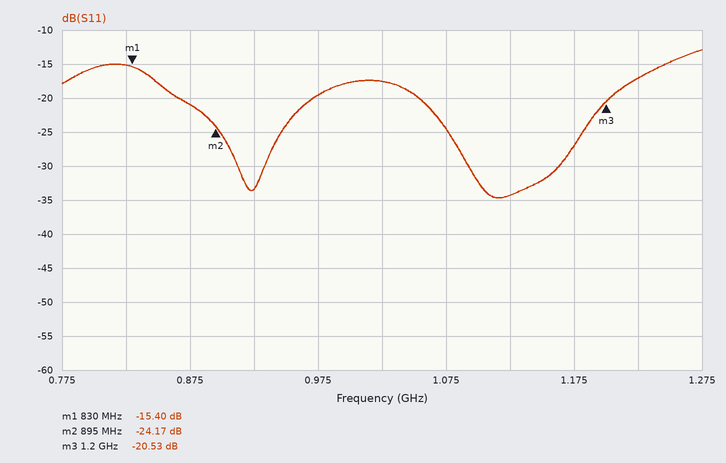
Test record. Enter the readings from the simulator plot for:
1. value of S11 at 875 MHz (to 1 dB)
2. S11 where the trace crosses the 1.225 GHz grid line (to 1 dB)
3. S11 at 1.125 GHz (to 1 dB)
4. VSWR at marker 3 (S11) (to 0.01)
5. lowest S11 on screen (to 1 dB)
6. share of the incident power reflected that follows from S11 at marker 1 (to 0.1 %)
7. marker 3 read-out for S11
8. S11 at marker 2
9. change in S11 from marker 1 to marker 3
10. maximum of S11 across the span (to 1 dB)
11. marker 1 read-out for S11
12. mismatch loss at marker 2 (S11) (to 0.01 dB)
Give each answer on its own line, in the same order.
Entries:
-21 dB
-17 dB
-34 dB
1.21
-35 dB
2.9 %
-20.53 dB
-24.17 dB
-5.13 dB
-13 dB
-15.40 dB
0.02 dB
